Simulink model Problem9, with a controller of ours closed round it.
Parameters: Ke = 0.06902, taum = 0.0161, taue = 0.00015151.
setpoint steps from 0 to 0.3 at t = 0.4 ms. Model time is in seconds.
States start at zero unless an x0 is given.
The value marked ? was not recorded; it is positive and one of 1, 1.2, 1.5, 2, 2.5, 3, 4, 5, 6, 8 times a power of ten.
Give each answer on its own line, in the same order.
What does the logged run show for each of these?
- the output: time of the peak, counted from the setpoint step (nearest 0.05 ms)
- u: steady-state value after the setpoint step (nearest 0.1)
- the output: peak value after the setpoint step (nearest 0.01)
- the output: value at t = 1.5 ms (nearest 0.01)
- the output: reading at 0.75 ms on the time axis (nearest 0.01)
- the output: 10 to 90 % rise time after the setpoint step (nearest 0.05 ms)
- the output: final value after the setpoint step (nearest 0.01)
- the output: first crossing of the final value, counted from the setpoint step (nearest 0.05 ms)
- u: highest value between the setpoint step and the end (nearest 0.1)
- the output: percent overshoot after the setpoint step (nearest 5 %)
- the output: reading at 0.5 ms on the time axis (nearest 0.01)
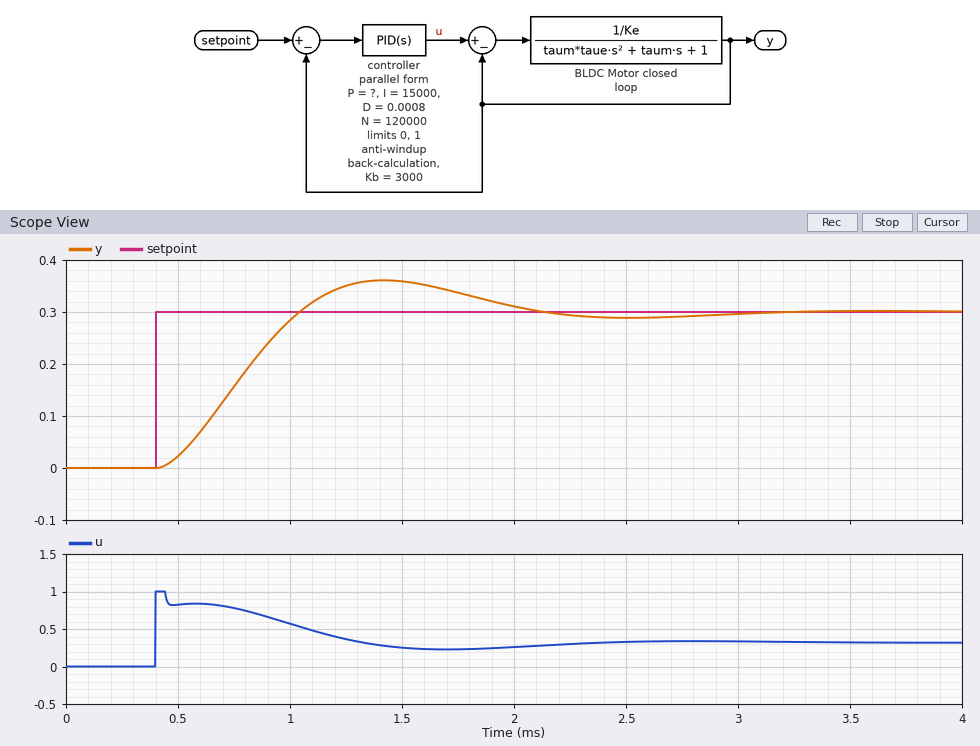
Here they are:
1.00 ms
0.3
0.36
0.36
0.16
0.45 ms
0.30
0.65 ms
1.0
20 %
0.02
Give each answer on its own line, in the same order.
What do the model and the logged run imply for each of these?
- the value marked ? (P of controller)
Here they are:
5
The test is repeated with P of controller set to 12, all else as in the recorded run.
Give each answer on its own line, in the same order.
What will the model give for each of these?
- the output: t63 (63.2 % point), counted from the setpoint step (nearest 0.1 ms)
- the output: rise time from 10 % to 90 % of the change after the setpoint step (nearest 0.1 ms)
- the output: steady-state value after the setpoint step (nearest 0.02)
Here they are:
0.4 ms
0.5 ms
0.30
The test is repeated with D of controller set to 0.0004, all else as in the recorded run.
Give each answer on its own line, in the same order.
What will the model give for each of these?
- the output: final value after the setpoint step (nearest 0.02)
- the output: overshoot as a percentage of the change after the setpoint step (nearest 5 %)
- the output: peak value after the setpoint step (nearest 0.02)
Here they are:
0.30
25 %
0.38
